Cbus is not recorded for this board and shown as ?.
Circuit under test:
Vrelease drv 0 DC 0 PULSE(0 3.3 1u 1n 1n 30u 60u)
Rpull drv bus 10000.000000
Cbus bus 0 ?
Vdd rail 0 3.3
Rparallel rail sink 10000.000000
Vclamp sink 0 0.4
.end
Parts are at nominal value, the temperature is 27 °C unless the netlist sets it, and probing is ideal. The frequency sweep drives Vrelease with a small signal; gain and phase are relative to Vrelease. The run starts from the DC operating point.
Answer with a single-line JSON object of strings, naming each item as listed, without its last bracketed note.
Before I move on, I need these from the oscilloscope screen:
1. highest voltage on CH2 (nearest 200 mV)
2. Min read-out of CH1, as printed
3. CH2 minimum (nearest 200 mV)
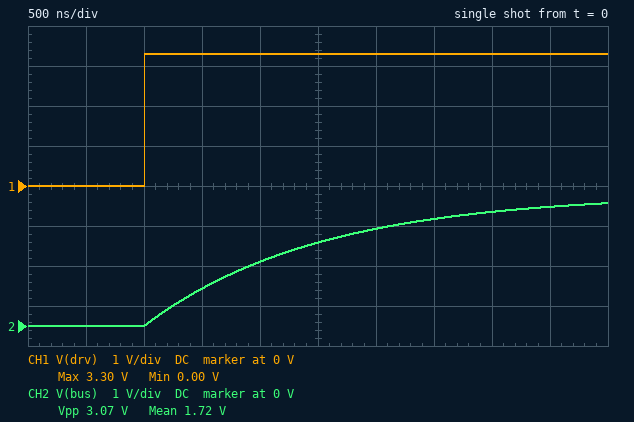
{"highest voltage on CH2": "3.0 V", "Min read-out of CH1, as printed": "0.00 V", "CH2 minimum": "0 V"}
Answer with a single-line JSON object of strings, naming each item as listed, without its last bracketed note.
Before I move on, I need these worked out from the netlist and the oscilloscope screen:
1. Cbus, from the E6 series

{"Cbus, from the E6 series": "150 pF"}
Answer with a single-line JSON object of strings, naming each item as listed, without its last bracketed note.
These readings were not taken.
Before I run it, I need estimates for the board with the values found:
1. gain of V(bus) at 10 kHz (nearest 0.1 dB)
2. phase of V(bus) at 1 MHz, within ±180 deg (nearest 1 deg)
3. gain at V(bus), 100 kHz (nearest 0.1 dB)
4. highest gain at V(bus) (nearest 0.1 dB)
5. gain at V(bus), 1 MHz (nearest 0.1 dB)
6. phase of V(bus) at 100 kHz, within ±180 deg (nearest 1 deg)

{"gain of V(bus) at 10 kHz": "0 dB", "phase of V(bus) at 1 MHz, within ±180 deg": "-84 deg", "gain at V(bus), 100 kHz": "-2.8 dB", "highest gain at V(bus)": "0 dB", "gain at V(bus), 1 MHz": "-19.5 dB", "phase of V(bus) at 100 kHz, within ±180 deg": "-43 deg"}
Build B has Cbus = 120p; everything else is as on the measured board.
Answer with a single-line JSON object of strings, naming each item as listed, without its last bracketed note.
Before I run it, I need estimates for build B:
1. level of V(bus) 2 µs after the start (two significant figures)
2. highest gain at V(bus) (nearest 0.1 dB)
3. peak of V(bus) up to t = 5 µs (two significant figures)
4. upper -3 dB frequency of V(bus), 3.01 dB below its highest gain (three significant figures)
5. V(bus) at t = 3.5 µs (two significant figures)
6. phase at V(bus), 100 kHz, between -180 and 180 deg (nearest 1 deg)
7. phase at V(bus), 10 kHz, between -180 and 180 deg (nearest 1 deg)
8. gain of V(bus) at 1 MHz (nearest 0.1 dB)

{"level of V(bus) 2 µs after the start": "1.9 V", "highest gain at V(bus)": "0 dB", "peak of V(bus) up to t = 5 µs": "3.2 V", "upper -3 dB frequency of V(bus), 3.01 dB below its highest gain": "133 kHz", "V(bus) at t = 3.5 µs": "2.9 V", "phase at V(bus), 100 kHz, between -180 and 180 deg": "-37 deg", "phase at V(bus), 10 kHz, between -180 and 180 deg": "-4 deg", "gain of V(bus) at 1 MHz": "-17.6 dB"}
